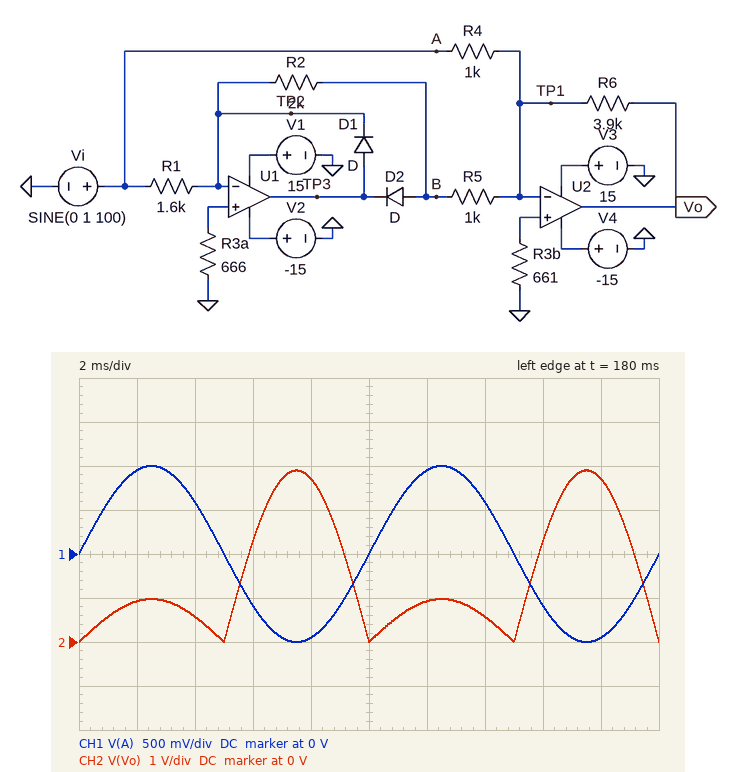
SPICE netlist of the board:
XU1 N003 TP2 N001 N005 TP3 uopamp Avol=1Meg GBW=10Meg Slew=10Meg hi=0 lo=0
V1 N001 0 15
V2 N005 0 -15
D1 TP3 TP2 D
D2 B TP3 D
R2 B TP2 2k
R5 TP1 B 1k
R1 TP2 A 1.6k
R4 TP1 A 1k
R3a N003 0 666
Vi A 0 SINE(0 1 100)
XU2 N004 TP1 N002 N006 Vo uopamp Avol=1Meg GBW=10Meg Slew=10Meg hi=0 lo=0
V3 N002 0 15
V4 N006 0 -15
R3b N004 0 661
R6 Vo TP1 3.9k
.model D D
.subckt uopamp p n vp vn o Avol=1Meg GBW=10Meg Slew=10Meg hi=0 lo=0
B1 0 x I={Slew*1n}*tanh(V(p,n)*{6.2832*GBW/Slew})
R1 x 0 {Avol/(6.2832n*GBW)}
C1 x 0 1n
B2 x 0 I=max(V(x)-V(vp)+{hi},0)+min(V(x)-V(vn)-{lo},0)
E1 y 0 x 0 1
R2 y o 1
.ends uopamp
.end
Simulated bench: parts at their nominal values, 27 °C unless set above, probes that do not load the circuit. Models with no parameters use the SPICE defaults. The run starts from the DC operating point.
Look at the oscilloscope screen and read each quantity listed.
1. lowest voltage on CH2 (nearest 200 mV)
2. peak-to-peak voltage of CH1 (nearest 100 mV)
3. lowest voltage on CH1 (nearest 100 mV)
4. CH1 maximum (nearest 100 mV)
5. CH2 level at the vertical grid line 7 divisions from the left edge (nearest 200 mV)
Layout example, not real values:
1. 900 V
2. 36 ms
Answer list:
1. 0 V
2. 2.0 V
3. -1.0 V
4. 1.0 V
5. 600 mV
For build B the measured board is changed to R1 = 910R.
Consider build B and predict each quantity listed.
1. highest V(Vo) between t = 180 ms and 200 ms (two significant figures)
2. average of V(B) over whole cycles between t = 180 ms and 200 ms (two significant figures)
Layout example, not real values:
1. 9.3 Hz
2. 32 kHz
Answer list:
1. 4.7 V
2. -700 mV
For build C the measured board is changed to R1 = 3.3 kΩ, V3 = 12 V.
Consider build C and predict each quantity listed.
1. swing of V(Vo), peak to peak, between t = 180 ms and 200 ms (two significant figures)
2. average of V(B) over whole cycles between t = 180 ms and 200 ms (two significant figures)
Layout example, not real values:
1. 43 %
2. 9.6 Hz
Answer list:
1. 5.4 V
2. -190 mV
